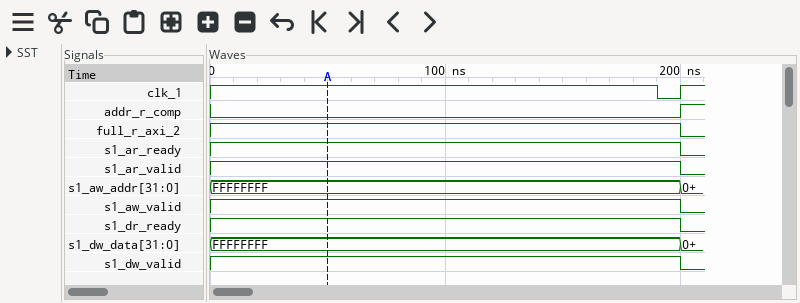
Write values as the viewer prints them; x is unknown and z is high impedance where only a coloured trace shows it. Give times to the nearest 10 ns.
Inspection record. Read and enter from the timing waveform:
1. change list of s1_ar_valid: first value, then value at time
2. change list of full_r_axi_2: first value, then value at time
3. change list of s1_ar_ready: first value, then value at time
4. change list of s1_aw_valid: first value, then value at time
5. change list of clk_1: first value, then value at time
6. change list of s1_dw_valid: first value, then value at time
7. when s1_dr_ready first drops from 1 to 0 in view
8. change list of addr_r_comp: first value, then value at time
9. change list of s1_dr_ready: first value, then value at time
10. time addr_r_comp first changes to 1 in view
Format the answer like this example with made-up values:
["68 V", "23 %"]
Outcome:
["1, 0 at 200 ns", "1, 0 at 200 ns", "1, 0 at 200 ns", "1, 0 at 200 ns", "1, 0 at 190 ns, 1 at 200 ns", "1, 0 at 200 ns", "200 ns", "0, 1 at 200 ns", "1, 0 at 200 ns", "200 ns"]
